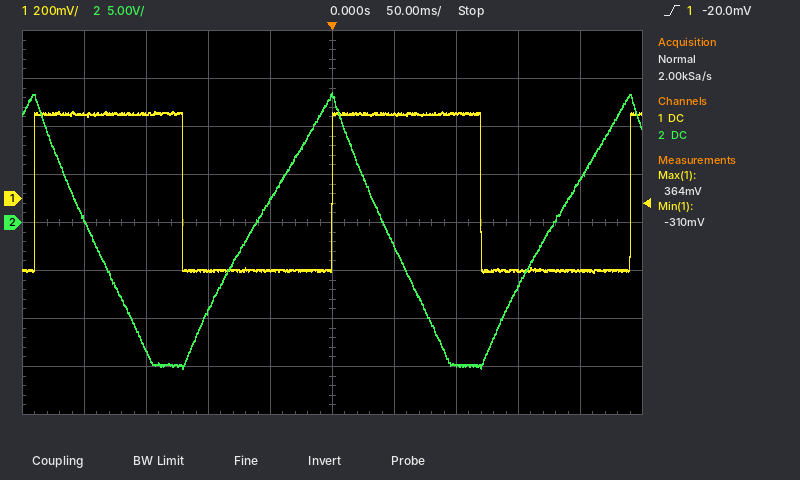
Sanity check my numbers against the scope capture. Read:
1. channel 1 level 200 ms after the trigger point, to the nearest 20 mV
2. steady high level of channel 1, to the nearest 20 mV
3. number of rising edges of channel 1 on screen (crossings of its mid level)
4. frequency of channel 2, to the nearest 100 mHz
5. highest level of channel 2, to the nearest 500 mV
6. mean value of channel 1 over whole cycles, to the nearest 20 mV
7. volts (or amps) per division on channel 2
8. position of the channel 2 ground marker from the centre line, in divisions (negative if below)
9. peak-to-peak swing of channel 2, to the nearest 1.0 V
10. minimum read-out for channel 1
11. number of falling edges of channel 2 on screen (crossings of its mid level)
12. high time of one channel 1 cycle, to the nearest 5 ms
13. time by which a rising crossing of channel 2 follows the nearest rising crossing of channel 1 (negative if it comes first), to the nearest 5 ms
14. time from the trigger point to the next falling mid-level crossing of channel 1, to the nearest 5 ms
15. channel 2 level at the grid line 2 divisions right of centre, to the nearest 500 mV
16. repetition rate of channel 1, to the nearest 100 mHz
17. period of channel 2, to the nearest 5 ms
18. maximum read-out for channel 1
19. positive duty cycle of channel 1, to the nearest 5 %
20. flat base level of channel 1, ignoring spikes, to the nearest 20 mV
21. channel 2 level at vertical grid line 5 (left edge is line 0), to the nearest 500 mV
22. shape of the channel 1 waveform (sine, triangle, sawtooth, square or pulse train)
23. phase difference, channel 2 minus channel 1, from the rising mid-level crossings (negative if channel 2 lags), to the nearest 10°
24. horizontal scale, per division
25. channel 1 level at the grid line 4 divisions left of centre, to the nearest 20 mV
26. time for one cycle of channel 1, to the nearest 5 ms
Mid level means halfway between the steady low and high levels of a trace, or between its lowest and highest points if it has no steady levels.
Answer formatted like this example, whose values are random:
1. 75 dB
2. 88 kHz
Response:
1. -300 mV
2. 360 mV
3. 3
4. 4.2 Hz
5. 13.5 V
6. 20 mV
7. 5 V
8. 0.0 div
9. 29.0 V
10. -310 mV
11. 2
12. 120 ms
13. -65 ms
14. 120 ms
15. -15.0 V
16. 4.2 Hz
17. 240 ms
18. 364 mV
19. 50 %
20. -300 mV
21. 13.0 V
22. square
23. +100°
24. 50 ms
25. 360 mV
26. 240 ms
